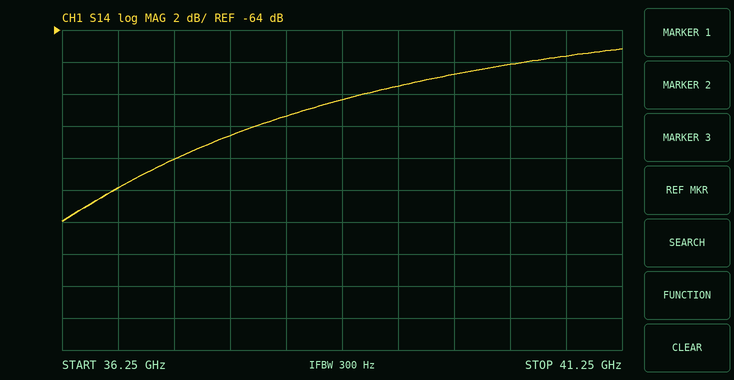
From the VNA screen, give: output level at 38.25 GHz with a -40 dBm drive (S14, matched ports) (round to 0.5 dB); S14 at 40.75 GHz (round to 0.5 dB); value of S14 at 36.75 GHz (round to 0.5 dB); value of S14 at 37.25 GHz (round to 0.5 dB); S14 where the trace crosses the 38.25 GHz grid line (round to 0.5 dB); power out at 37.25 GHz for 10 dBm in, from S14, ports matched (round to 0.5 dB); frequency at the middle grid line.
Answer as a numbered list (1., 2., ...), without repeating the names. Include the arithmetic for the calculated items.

1. -40 dBm + (-69.5 dB) = -109.5 dBm
2. -65.5 dB
3. -74.0 dB
4. -72.0 dB
5. -69.5 dB
6. 10 dBm + (-72.0 dB) = -62.0 dBm
7. 38.75 GHz
